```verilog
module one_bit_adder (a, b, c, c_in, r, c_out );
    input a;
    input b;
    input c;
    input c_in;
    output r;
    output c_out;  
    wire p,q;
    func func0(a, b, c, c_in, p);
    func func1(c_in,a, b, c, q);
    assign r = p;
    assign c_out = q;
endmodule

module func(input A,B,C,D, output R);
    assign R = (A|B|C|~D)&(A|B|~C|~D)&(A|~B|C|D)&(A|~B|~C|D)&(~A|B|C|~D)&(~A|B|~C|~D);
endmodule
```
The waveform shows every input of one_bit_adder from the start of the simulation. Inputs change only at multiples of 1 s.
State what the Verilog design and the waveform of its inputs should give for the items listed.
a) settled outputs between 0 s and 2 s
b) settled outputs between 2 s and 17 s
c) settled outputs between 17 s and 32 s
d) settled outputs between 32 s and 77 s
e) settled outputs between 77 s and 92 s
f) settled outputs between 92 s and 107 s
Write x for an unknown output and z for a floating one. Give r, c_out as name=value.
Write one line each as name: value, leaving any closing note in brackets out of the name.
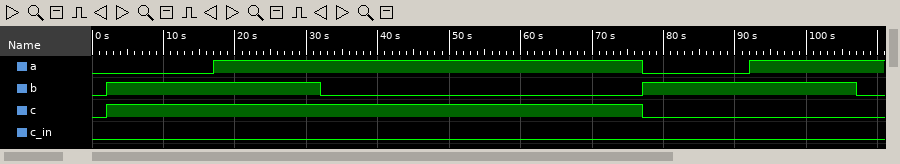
settled outputs between 0 s and 2 s: r=1, c_out=1
settled outputs between 2 s and 17 s: r=0, c_out=0
settled outputs between 17 s and 32 s: r=1, c_out=1
settled outputs between 32 s and 77 s: r=1, c_out=1
settled outputs between 77 s and 92 s: r=0, c_out=1
settled outputs between 92 s and 107 s: r=1, c_out=0
